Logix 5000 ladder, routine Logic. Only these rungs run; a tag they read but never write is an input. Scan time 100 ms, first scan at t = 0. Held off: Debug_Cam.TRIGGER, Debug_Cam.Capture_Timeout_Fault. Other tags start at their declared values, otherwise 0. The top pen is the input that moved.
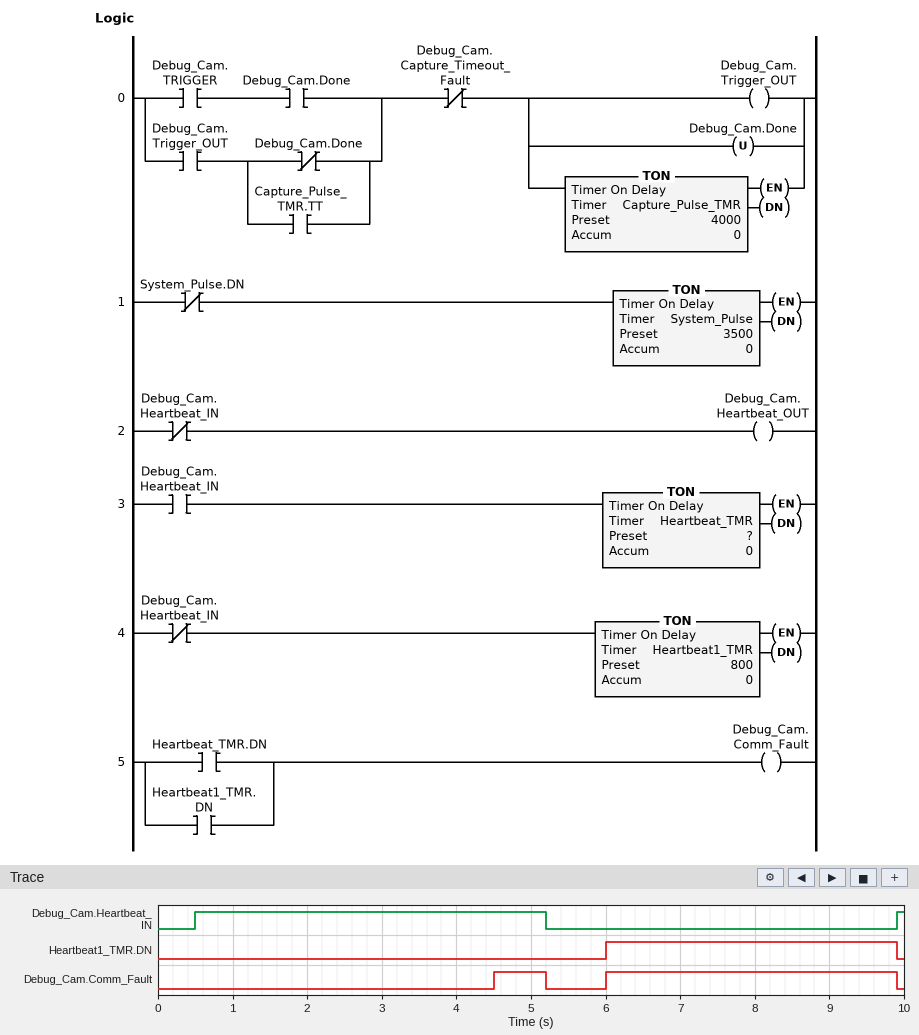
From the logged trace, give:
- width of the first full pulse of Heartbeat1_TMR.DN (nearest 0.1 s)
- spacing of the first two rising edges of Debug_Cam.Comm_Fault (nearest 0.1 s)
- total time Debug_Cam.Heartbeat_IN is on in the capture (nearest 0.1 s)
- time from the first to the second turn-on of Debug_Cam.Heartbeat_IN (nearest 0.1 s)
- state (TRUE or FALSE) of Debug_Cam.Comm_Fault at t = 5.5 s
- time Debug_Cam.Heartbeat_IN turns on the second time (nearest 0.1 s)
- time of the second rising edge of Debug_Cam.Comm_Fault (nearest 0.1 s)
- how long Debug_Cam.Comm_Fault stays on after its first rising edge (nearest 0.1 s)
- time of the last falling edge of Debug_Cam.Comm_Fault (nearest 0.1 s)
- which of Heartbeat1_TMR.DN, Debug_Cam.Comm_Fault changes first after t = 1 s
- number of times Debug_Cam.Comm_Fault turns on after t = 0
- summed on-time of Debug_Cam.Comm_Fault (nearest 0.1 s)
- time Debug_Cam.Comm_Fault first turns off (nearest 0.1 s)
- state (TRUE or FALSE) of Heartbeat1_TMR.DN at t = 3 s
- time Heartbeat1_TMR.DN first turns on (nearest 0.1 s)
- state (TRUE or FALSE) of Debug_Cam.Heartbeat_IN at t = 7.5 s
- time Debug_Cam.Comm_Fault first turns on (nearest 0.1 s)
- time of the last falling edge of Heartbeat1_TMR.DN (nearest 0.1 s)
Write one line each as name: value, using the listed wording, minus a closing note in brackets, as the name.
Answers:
width of the first full pulse of Heartbeat1_TMR.DN: 3.9 s
spacing of the first two rising edges of Debug_Cam.Comm_Fault: 1.5 s
total time Debug_Cam.Heartbeat_IN is on in the capture: 4.8 s
time from the first to the second turn-on of Debug_Cam.Heartbeat_IN: 9.4 s
state (TRUE or FALSE) of Debug_Cam.Comm_Fault at t = 5.5 s: FALSE
time Debug_Cam.Heartbeat_IN turns on the second time: 9.9 s
time of the second rising edge of Debug_Cam.Comm_Fault: 6.0 s
how long Debug_Cam.Comm_Fault stays on after its first rising edge: 0.7 s
time of the last falling edge of Debug_Cam.Comm_Fault: 9.9 s
which of Heartbeat1_TMR.DN, Debug_Cam.Comm_Fault changes first after t = 1 s: Debug_Cam.Comm_Fault
number of times Debug_Cam.Comm_Fault turns on after t = 0: 2
summed on-time of Debug_Cam.Comm_Fault: 4.6 s
time Debug_Cam.Comm_Fault first turns off: 5.2 s
state (TRUE or FALSE) of Heartbeat1_TMR.DN at t = 3 s: FALSE
time Heartbeat1_TMR.DN first turns on: 6.0 s
state (TRUE or FALSE) of Debug_Cam.Heartbeat_IN at t = 7.5 s: FALSE
time Debug_Cam.Comm_Fault first turns on: 4.5 s
time of the last falling edge of Heartbeat1_TMR.DN: 9.9 s
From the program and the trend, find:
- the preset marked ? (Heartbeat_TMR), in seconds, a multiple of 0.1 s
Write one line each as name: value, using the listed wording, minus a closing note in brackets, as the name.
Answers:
the preset marked ? (Heartbeat_TMR), in seconds, a multiple of 0.1 s: 4.0 s
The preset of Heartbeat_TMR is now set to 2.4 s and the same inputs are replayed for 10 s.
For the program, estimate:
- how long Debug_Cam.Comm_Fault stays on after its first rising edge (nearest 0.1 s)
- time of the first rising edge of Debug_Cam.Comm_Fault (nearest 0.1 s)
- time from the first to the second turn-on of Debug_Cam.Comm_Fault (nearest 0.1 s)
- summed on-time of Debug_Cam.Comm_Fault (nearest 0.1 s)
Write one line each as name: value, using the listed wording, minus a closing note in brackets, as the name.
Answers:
how long Debug_Cam.Comm_Fault stays on after its first rising edge: 2.3 s
time of the first rising edge of Debug_Cam.Comm_Fault: 2.9 s
time from the first to the second turn-on of Debug_Cam.Comm_Fault: 3.1 s
summed on-time of Debug_Cam.Comm_Fault: 6.2 s
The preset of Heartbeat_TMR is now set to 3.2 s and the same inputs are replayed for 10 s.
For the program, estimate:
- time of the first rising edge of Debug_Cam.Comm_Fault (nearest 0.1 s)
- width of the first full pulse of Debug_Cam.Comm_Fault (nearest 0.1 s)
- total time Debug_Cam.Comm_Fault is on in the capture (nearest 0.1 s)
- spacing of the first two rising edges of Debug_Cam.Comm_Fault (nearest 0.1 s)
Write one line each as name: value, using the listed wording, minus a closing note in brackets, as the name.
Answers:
time of the first rising edge of Debug_Cam.Comm_Fault: 3.7 s
width of the first full pulse of Debug_Cam.Comm_Fault: 1.5 s
total time Debug_Cam.Comm_Fault is on in the capture: 5.4 s
spacing of the first two rising edges of Debug_Cam.Comm_Fault: 2.3 s
